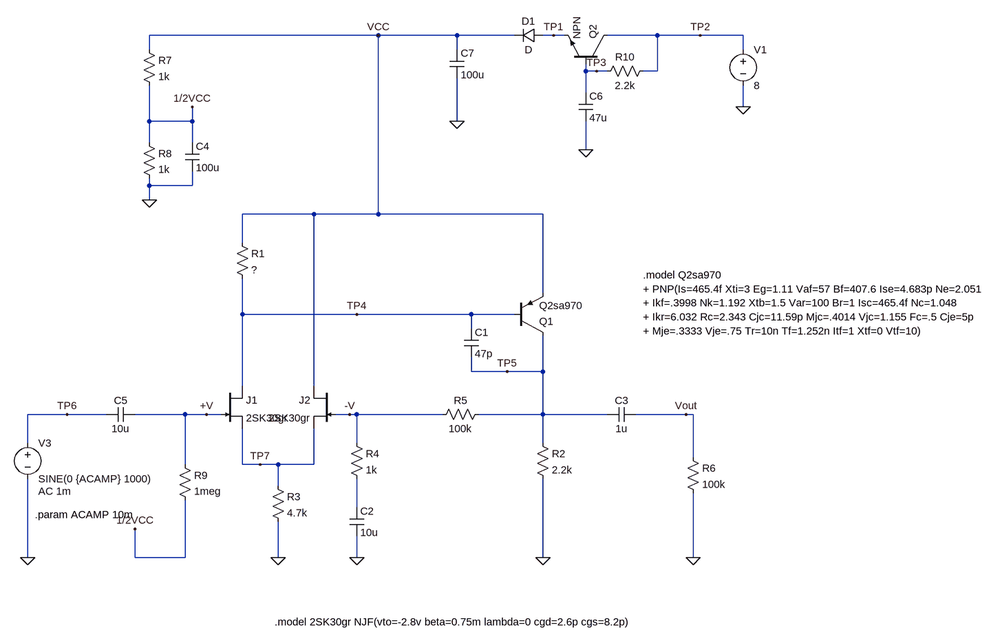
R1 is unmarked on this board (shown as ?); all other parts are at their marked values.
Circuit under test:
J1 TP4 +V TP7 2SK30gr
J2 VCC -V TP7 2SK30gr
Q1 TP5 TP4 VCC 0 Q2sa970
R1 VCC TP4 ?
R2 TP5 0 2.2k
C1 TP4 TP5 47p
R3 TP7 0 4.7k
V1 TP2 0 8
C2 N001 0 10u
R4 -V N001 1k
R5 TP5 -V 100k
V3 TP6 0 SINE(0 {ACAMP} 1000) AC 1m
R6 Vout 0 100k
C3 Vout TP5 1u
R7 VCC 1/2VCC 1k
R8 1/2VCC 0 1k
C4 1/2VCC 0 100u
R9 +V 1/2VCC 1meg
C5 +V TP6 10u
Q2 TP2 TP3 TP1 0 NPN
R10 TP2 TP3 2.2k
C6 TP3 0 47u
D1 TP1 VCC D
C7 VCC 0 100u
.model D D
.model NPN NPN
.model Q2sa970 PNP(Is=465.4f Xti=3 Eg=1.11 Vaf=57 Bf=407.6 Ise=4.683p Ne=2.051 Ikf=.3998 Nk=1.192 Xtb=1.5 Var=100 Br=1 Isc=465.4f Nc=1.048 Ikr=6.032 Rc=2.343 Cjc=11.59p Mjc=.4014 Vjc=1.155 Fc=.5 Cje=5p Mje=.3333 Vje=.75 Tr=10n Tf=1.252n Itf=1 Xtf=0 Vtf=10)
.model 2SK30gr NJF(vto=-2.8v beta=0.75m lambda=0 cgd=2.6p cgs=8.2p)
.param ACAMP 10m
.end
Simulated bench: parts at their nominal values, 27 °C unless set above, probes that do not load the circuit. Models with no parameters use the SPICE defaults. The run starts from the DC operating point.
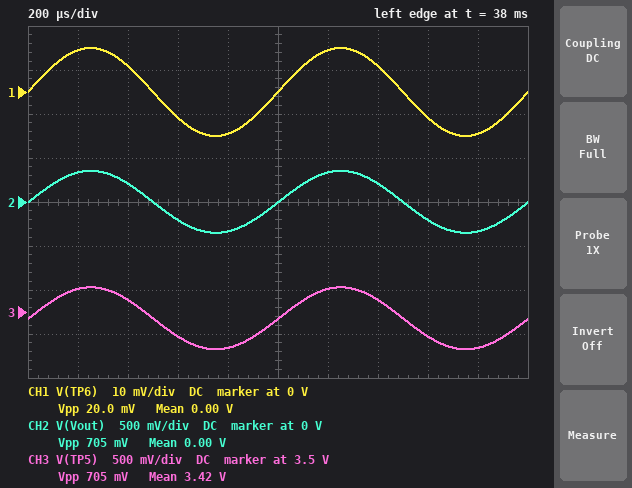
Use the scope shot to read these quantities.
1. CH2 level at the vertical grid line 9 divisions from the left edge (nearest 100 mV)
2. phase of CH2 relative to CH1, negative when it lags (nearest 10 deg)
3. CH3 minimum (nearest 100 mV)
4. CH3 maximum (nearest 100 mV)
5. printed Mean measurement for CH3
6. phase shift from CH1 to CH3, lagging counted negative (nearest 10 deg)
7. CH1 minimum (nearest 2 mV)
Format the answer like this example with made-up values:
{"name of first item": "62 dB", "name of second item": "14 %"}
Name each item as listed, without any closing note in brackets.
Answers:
{"CH2 level at the vertical grid line 9 divisions from the left edge": "-300 mV", "phase of CH2 relative to CH1, negative when it lags": "0 deg", "CH3 minimum": "3.1 V", "CH3 maximum": "3.8 V", "printed Mean measurement for CH3": "3.42 V", "phase shift from CH1 to CH3, lagging counted negative": "0 deg", "CH1 minimum": "-10 mV"}
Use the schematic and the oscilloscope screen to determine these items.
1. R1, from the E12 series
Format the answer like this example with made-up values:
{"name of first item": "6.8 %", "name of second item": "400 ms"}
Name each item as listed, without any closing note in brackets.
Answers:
{"R1, from the E12 series": "1.5 kΩ"}
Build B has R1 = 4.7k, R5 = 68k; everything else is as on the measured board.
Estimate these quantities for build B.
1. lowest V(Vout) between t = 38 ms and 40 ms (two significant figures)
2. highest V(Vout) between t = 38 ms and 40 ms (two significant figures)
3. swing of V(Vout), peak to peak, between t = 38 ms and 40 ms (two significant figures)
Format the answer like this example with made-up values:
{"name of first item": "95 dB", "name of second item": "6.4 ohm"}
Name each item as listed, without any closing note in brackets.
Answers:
{"lowest V(Vout) between t = 38 ms and 40 ms": "-330 mV", "highest V(Vout) between t = 38 ms and 40 ms": "320 mV", "swing of V(Vout), peak to peak, between t = 38 ms and 40 ms": "650 mV"}
